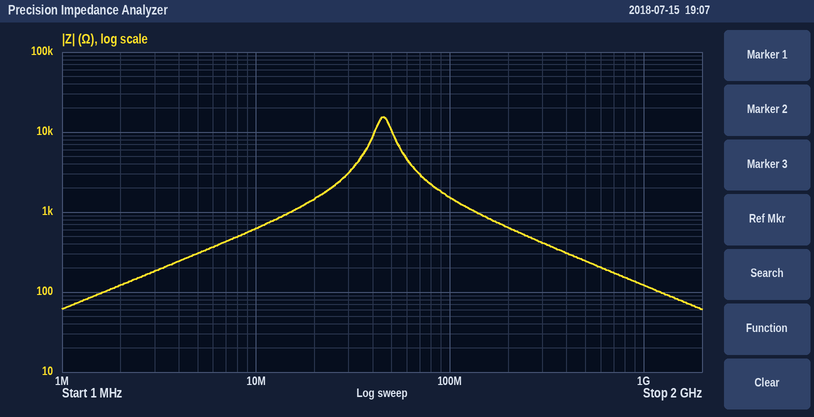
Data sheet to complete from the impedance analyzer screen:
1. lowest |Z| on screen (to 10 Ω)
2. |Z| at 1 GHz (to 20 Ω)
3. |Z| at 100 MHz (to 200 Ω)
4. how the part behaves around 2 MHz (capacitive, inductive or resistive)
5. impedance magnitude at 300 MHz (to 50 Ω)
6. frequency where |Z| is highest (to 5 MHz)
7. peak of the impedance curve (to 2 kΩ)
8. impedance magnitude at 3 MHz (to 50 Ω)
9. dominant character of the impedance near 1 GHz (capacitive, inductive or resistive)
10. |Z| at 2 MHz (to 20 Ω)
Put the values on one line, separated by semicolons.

60 Ω; 120 Ω; 1.6 kΩ; inductive; 400 Ω; 45 MHz; 16 kΩ; 200 Ω; capacitive; 120 Ω
